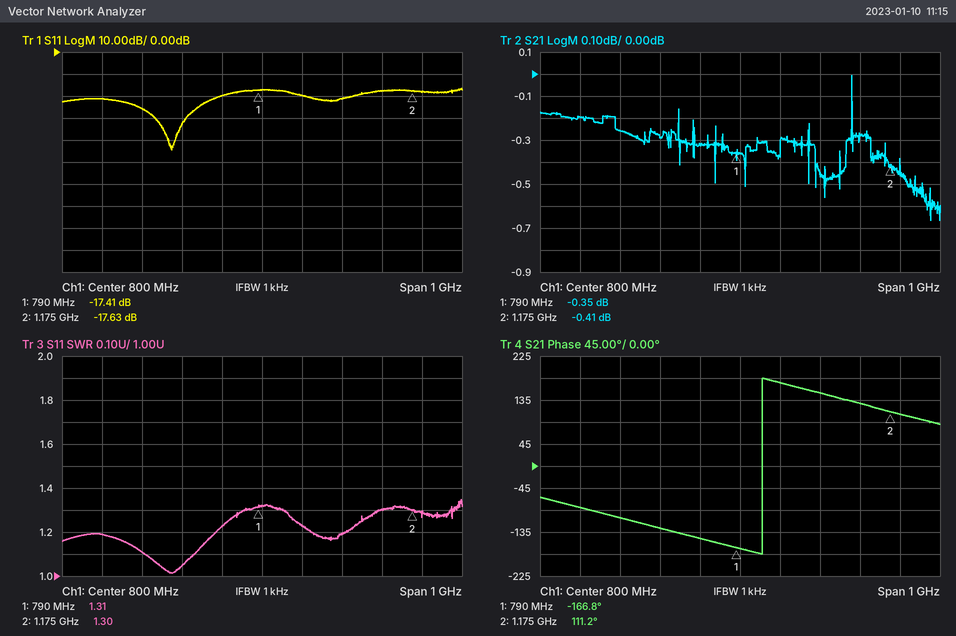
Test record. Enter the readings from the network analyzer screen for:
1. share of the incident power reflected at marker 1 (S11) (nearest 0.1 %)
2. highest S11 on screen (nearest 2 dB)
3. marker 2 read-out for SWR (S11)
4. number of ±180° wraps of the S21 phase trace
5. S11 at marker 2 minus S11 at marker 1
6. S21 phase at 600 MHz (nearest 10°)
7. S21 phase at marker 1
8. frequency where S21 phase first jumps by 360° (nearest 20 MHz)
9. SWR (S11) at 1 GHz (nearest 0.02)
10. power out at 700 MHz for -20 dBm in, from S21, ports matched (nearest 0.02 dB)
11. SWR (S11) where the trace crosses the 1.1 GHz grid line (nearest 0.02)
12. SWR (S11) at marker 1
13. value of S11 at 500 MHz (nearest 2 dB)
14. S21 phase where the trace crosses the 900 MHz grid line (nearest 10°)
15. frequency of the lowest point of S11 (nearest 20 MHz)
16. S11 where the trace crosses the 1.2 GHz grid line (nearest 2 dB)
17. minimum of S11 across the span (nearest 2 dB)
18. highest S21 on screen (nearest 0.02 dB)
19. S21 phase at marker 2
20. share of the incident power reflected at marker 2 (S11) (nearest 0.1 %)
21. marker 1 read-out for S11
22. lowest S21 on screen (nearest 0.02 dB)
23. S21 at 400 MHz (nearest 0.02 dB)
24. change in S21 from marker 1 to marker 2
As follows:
1.8 %
-16 dB
1.30
1
-0.22 dB
-130°
-166.8°
860 MHz
1.20
-20.32 dBm
1.30
1.31
-26 dB
170°
580 MHz
-18 dB
-44 dB
0.00 dB
111.2°
1.7 %
-17.41 dB
-0.66 dB
-0.20 dB
-0.06 dB
